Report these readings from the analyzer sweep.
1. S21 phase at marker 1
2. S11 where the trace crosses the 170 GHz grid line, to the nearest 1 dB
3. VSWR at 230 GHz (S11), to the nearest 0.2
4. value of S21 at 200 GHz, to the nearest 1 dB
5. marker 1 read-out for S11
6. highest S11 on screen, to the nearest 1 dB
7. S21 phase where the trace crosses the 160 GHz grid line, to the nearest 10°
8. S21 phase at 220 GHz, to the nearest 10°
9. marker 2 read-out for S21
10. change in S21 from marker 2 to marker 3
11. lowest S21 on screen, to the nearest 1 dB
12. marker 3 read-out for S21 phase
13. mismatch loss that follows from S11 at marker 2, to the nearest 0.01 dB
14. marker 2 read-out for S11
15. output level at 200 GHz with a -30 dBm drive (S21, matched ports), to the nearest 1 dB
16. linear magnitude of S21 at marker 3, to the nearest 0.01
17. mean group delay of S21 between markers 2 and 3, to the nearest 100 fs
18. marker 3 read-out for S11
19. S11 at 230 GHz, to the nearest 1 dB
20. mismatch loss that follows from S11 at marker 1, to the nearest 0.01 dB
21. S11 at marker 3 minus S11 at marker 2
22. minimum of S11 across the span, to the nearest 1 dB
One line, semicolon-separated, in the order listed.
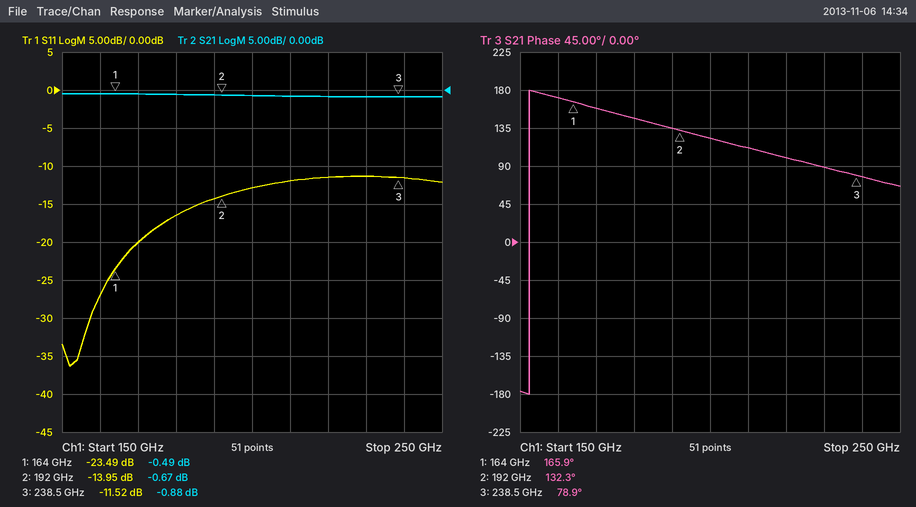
165.9°; -20 dB; 1.8; -1 dB; -23.49 dB; -11 dB; 170°; 100°; -0.67 dB; -0.21 dB; -1 dB; 78.9°; 0.18 dB; -13.95 dB; -31 dBm; 0.90; 3.2 ps; -11.52 dB; -11 dB; 0.02 dB; 2.43 dB; -36 dB
